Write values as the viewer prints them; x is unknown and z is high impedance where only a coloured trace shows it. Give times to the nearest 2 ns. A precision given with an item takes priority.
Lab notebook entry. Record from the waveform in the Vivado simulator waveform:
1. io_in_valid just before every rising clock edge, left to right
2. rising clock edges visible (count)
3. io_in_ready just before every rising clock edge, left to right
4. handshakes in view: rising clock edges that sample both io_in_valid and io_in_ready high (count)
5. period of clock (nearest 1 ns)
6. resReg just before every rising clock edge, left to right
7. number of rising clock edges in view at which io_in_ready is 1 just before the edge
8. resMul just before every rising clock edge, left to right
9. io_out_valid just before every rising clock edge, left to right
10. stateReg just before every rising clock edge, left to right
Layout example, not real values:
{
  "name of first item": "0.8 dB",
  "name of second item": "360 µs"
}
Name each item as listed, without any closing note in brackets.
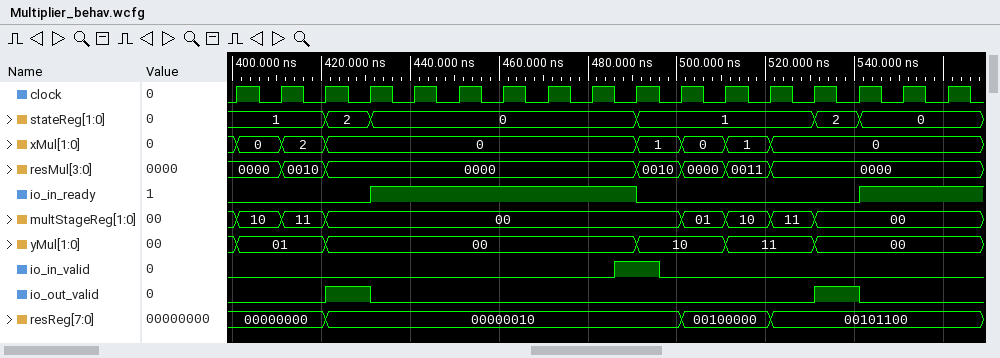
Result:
{
  "io_in_valid just before every rising clock edge, left to right": "0 0 0 0 0 0 0 0 0 1 0 0 0 0 0 0 0",
  "rising clock edges visible": "17",
  "io_in_ready just before every rising clock edge, left to right": "0 0 0 0 1 1 1 1 1 1 0 0 0 0 0 1 1",
  "handshakes in view: rising clock edges that sample both io_in_valid and io_in_ready high": "1",
  "period of clock": "10 ns",
  "resReg just before every rising clock edge, left to right": "00000000, 00000000, 00000000, 00000010, 00000010, 00000010, 00000010, 00000010, 00000010, 00000010, 00000010, 00100000, 00100000, 00101100, 00101100, 00101100, 00101100",
  "number of rising clock edges in view at which io_in_ready is 1 just before the edge": "8",
  "resMul just before every rising clock edge, left to right": "0000, 0000, 0010, 0000, 0000, 0000, 0000, 0000, 0000, 0000, 0010, 0000, 0011, 0000, 0000, 0000, 0000",
  "io_out_valid just before every rising clock edge, left to right": "0 0 0 1 0 0 0 0 0 0 0 0 0 0 1 0 0",
  "stateReg just before every rising clock edge, left to right": "1, 1, 1, 2, 0, 0, 0, 0, 0, 0, 1, 1, 1, 1, 2, 0, 0"
}
